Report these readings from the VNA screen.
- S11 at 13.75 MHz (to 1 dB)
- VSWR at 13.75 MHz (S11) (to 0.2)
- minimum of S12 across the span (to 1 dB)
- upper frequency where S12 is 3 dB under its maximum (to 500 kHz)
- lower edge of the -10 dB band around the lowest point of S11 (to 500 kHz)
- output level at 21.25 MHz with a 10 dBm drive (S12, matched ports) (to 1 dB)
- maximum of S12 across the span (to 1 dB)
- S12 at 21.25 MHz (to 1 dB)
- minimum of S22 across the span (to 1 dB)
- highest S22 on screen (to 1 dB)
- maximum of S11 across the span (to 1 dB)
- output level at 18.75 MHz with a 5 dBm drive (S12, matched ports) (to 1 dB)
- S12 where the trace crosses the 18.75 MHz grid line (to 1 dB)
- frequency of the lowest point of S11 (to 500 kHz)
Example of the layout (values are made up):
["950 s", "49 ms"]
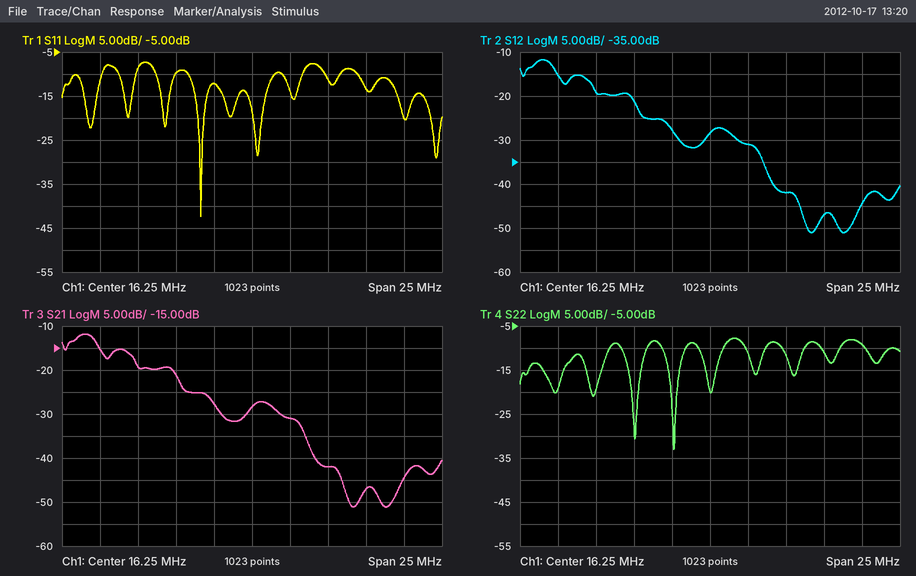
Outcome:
["-12 dB", "1.6", "-51 dB", "6.0 MHz", "12.0 MHz", "-32 dBm", "-12 dB", "-42 dB", "-33 dB", "-8 dB", "-7 dB", "-26 dBm", "-31 dB", "13.0 MHz"]
